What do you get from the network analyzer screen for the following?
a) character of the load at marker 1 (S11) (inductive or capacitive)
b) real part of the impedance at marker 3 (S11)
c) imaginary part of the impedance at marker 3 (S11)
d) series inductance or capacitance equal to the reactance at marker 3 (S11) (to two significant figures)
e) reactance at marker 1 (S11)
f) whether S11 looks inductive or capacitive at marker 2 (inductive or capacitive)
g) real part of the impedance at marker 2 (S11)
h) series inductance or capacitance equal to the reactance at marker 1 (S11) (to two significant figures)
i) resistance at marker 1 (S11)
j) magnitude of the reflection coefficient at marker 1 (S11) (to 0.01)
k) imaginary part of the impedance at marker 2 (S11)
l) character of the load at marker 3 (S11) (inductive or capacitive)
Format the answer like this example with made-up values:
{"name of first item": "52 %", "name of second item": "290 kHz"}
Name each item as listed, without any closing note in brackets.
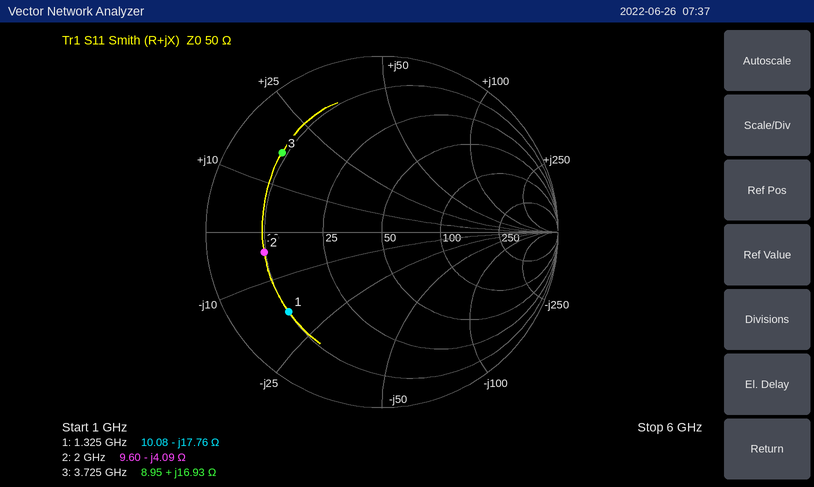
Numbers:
{"character of the load at marker 1 (S11)": "capacitive", "real part of the impedance at marker 3": "8.95 Ω", "imaginary part of the impedance at marker 3": "+16.93 Ω", "series inductance or capacitance equal to the reactance at marker 3 (S11)": "720 pH", "reactance at marker 1": "-17.76 Ω", "whether S11 looks inductive or capacitive at marker 2": "capacitive", "real part of the impedance at marker 2": "9.60 Ω", "series inductance or capacitance equal to the reactance at marker 1 (S11)": "6.8 pF", "resistance at marker 1": "10.08 Ω", "magnitude of the reflection coefficient at marker 1 (S11)": "0.70", "imaginary part of the impedance at marker 2": "-4.09 Ω", "character of the load at marker 3 (S11)": "inductive"}
